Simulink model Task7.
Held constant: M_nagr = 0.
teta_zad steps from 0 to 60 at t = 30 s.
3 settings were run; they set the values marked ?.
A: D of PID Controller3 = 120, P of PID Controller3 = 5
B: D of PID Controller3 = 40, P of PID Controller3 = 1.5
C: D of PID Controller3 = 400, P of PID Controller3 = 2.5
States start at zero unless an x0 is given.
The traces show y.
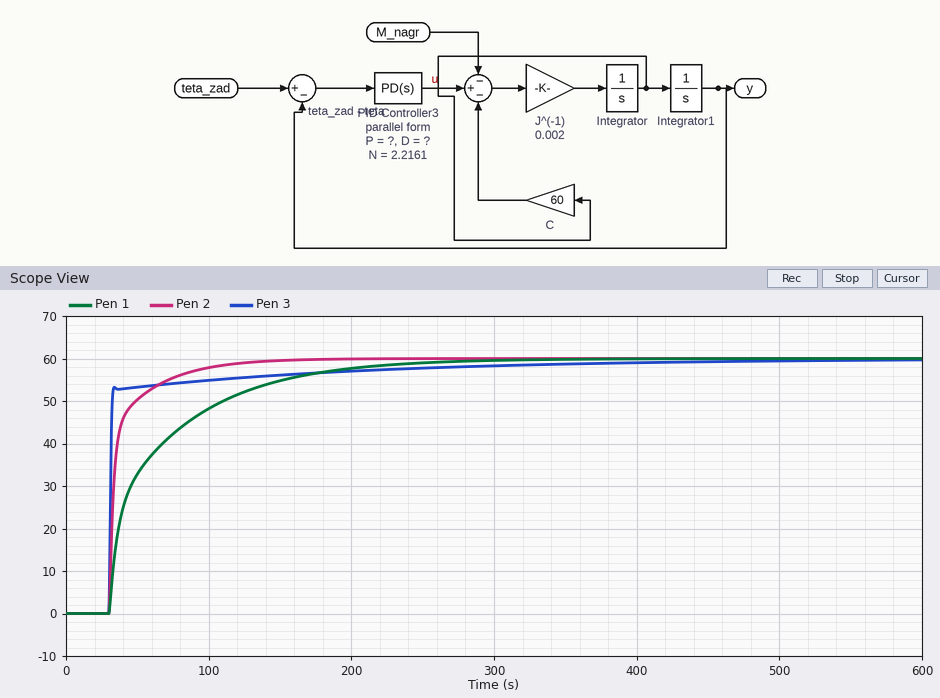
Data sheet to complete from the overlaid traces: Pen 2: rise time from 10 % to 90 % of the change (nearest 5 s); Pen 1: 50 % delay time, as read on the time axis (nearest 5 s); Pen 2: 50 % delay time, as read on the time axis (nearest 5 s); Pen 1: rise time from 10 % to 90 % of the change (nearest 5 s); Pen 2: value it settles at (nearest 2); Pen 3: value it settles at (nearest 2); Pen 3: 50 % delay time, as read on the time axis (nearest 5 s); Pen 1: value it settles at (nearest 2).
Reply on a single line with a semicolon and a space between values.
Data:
35 s; 45 s; 35 s; 110 s; 60; 60; 30 s; 60
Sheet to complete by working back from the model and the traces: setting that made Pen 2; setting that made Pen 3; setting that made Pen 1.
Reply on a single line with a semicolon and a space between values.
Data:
A; C; B
